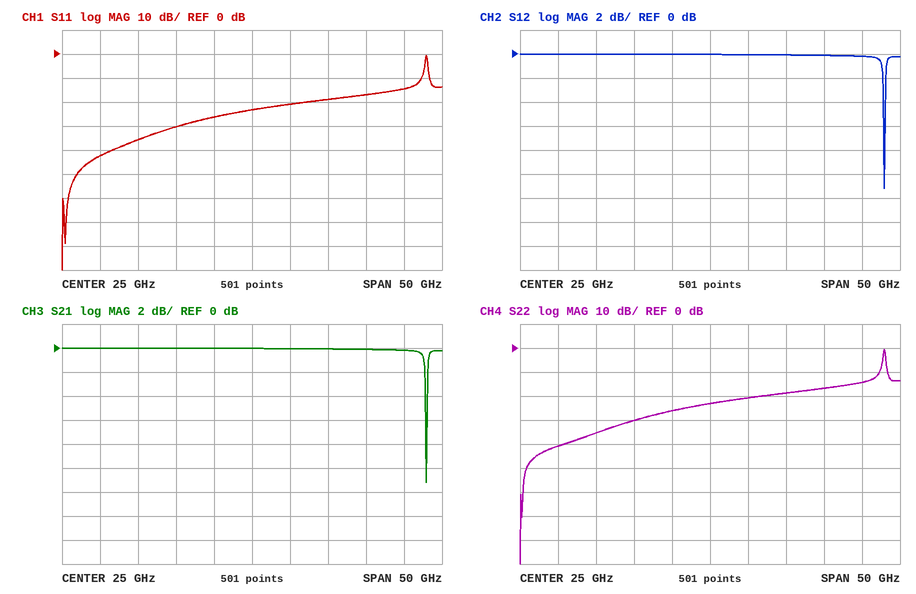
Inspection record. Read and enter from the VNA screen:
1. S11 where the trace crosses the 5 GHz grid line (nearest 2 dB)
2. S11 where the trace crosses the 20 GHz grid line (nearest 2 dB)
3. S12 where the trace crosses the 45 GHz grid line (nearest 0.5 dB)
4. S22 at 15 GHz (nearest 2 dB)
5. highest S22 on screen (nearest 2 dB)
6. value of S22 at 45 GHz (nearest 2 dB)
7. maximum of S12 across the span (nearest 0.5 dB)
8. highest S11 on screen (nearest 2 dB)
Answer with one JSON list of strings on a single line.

["-42 dB", "-26 dB", "0.0 dB", "-30 dB", "0 dB", "-14 dB", "0.0 dB", "0 dB"]
